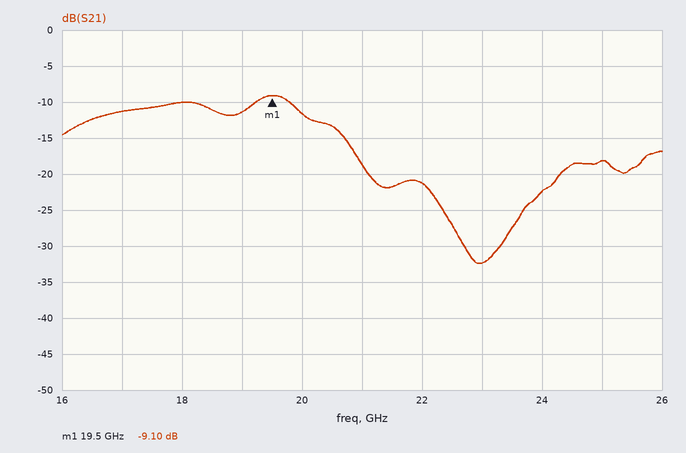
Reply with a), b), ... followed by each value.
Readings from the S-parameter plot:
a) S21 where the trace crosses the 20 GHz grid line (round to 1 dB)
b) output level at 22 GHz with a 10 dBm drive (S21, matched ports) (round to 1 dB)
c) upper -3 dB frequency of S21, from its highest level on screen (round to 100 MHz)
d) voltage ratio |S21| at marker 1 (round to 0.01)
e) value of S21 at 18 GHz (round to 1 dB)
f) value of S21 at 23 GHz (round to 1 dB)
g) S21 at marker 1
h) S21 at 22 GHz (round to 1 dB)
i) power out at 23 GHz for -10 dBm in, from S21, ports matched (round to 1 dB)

a) -12 dB
b) -11 dBm
c) 20.1 GHz
d) 0.35
e) -10 dB
f) -32 dB
g) -9.10 dB
h) -21 dB
i) -42 dBm
